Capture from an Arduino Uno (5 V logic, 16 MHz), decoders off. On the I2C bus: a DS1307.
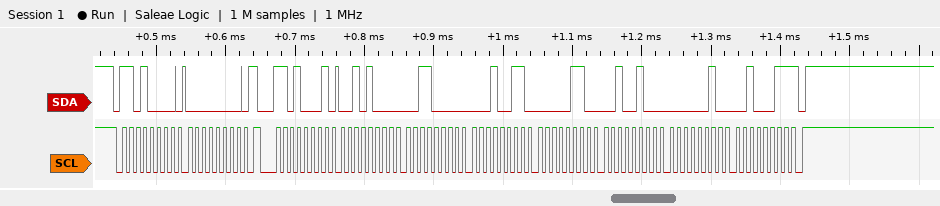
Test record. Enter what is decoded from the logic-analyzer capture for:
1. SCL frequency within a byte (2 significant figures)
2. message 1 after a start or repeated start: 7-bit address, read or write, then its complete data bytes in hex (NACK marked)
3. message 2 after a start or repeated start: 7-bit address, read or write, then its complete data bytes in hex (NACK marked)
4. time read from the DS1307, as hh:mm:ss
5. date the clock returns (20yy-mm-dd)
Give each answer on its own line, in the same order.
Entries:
100 kHz
0x68 write: 00
0x68 read: 28 30 13 06 24 02 23 NACK
13:30:28
2023-02-24
